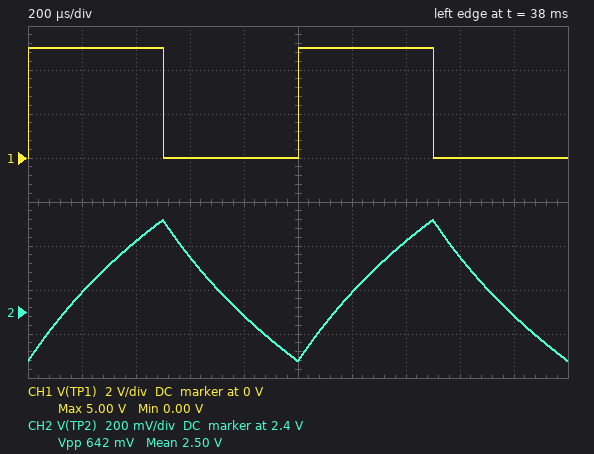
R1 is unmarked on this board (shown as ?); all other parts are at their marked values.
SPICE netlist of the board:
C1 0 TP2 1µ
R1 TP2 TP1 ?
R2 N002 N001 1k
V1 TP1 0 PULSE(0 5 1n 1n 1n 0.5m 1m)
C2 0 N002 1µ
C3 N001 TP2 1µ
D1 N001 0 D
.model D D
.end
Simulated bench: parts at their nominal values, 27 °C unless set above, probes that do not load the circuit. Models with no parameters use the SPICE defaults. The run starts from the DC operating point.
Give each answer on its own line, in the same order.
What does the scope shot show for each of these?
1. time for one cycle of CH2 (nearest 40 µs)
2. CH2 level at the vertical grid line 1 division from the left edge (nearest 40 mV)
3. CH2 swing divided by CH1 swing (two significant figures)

1.00 ms
2.48 V
0.13
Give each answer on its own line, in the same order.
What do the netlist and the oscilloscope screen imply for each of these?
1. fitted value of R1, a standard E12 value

1.8 kΩ
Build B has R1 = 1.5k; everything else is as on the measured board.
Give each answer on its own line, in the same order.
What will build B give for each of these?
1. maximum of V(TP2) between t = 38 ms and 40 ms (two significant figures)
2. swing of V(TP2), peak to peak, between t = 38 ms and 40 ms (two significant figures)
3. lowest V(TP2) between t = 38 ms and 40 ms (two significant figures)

2.9 V
770 mV
2.1 V
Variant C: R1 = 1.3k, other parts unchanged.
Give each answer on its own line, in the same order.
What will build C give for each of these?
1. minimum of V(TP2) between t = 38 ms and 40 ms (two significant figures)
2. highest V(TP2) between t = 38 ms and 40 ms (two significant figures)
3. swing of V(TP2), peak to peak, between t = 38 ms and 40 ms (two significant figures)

2.1 V
2.9 V
880 mV
